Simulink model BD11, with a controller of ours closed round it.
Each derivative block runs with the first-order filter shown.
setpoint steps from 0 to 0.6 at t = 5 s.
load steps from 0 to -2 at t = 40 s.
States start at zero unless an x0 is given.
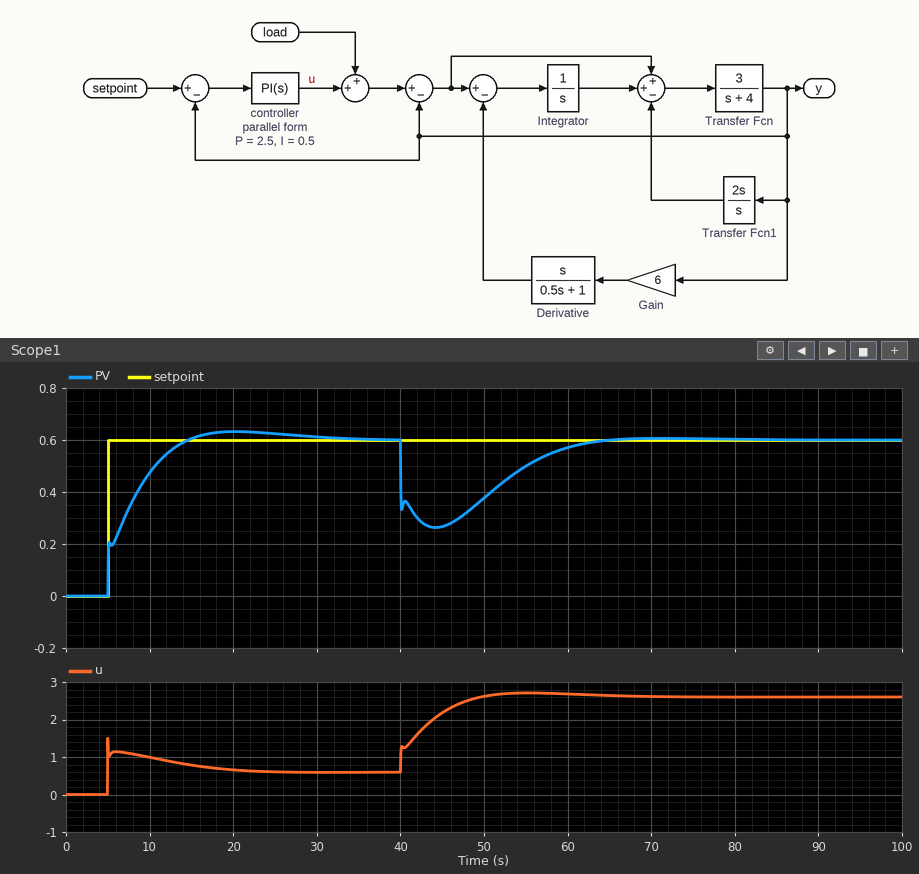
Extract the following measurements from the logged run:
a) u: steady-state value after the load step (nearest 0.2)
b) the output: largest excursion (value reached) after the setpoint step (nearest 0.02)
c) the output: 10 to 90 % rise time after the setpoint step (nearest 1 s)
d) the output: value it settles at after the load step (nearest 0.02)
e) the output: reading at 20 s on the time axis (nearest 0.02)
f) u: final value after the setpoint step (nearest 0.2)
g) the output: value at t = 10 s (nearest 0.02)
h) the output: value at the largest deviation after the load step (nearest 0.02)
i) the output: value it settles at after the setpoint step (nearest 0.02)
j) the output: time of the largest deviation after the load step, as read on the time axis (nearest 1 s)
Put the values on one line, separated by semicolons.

2.6; 0.64; 7 s; 0.60; 0.64; 0.6; 0.48; 0.26; 0.60; 44 s
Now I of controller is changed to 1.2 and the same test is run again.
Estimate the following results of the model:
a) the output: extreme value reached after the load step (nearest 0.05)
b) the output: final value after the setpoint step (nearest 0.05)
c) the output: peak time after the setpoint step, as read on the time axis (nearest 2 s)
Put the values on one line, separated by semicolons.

0.35; 0.60; 14 s
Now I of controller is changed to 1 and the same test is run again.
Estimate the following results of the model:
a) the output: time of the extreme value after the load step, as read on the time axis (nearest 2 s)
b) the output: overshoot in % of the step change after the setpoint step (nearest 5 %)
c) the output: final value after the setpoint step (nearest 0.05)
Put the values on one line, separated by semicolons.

42 s; 10 %; 0.60
